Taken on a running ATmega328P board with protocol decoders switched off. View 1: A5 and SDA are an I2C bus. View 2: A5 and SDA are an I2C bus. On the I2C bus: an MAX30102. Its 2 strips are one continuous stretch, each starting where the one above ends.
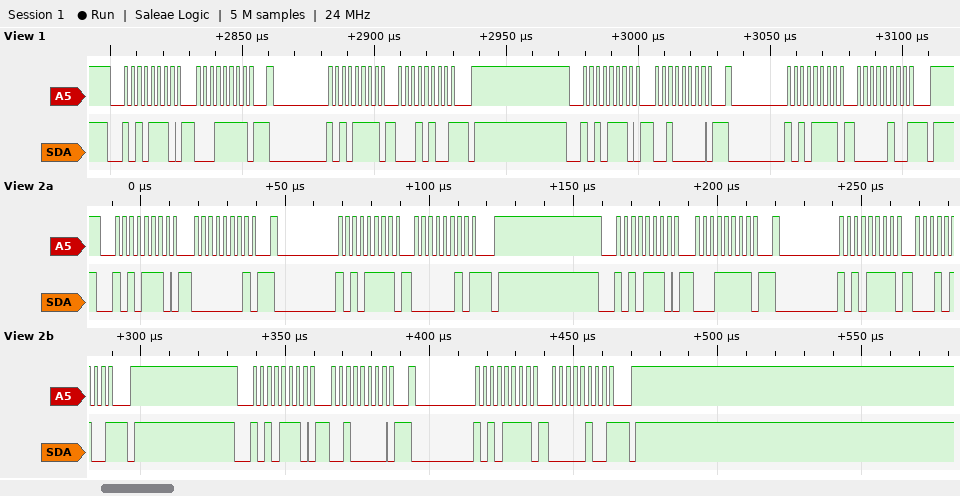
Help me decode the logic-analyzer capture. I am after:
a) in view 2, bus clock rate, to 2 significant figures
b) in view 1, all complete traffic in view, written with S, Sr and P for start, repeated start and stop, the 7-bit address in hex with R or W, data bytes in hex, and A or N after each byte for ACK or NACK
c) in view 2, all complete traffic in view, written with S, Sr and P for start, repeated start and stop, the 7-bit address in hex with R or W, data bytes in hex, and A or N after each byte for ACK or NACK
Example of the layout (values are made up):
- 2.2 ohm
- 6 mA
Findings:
- 400 kHz
- S 57W A 1F A Sr 57R A 14 N P S 57W A 20 A Sr 57R A 04 N P
- S 57W A 01 A Sr 57R A 02 N P S 57W A 1F A Sr 57R A 14 N P S 57W A 20 A Sr 57R A 04 N P
